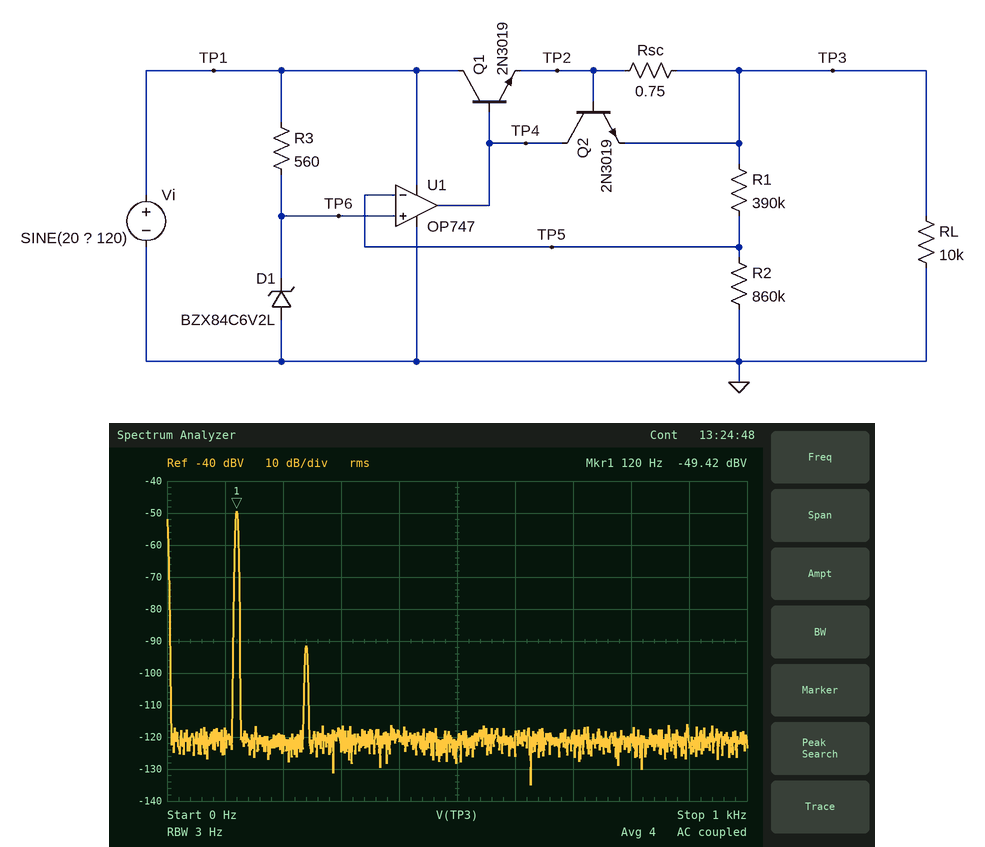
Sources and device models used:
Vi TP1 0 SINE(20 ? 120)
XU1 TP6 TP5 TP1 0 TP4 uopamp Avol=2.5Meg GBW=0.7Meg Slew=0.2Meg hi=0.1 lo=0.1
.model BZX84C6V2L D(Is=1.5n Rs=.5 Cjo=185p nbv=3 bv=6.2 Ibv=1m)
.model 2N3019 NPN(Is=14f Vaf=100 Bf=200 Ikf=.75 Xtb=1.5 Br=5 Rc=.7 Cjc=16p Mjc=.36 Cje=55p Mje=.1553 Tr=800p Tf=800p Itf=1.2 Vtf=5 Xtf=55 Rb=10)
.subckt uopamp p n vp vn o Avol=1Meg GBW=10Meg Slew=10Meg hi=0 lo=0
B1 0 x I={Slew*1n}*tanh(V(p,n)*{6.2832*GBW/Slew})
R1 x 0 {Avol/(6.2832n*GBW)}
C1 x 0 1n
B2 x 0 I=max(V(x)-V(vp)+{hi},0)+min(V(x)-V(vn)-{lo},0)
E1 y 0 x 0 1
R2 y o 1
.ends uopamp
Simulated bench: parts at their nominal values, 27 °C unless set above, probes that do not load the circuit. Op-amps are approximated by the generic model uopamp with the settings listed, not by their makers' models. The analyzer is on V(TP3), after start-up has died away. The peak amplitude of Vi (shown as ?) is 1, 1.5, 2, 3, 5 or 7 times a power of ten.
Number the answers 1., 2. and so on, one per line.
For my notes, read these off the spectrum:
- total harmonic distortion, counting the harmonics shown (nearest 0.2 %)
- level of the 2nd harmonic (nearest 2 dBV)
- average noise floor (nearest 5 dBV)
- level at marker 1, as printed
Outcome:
1. 0.8 %
2. -92 dBV
3. -120 dBV
4. -49.42 dBV
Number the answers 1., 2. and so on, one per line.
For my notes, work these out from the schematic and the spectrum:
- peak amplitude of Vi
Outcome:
1. 500 mV
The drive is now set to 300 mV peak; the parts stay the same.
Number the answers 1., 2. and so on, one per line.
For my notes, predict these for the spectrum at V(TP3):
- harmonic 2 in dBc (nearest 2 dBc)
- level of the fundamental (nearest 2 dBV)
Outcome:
1. -46 dBc
2. -54 dBV
